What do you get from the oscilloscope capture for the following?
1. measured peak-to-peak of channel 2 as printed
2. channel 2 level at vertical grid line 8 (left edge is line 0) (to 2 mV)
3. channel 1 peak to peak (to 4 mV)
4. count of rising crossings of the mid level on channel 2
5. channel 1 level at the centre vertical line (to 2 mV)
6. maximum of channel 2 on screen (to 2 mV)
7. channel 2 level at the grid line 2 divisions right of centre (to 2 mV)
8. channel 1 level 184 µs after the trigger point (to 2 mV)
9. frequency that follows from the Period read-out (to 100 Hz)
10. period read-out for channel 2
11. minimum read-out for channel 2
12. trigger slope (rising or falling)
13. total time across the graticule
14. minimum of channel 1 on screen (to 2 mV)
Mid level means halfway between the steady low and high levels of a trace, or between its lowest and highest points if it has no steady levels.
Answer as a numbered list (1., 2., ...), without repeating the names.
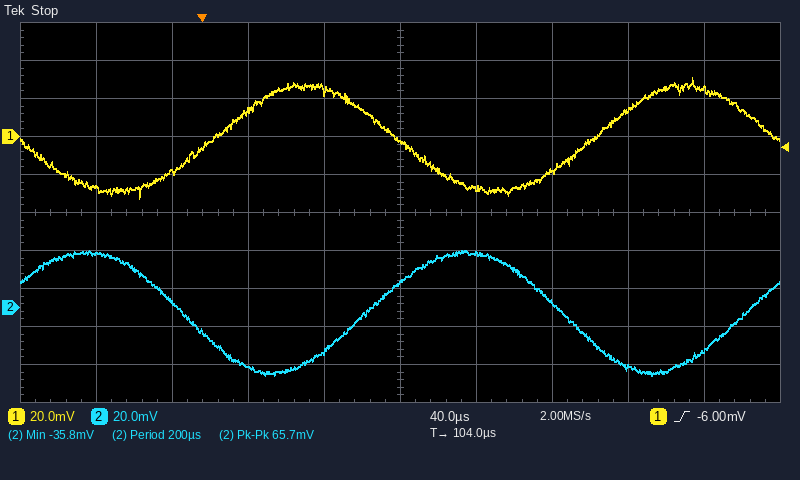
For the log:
1. 65.7 mV
2. -32 mV
3. 64 mV
4. 2
5. -2 mV
6. 30 mV
7. 2 mV
8. -18 mV
9. 5.0 kHz
10. 200 µs
11. -35.8 mV
12. rising
13. 400 µs
14. -32 mV
